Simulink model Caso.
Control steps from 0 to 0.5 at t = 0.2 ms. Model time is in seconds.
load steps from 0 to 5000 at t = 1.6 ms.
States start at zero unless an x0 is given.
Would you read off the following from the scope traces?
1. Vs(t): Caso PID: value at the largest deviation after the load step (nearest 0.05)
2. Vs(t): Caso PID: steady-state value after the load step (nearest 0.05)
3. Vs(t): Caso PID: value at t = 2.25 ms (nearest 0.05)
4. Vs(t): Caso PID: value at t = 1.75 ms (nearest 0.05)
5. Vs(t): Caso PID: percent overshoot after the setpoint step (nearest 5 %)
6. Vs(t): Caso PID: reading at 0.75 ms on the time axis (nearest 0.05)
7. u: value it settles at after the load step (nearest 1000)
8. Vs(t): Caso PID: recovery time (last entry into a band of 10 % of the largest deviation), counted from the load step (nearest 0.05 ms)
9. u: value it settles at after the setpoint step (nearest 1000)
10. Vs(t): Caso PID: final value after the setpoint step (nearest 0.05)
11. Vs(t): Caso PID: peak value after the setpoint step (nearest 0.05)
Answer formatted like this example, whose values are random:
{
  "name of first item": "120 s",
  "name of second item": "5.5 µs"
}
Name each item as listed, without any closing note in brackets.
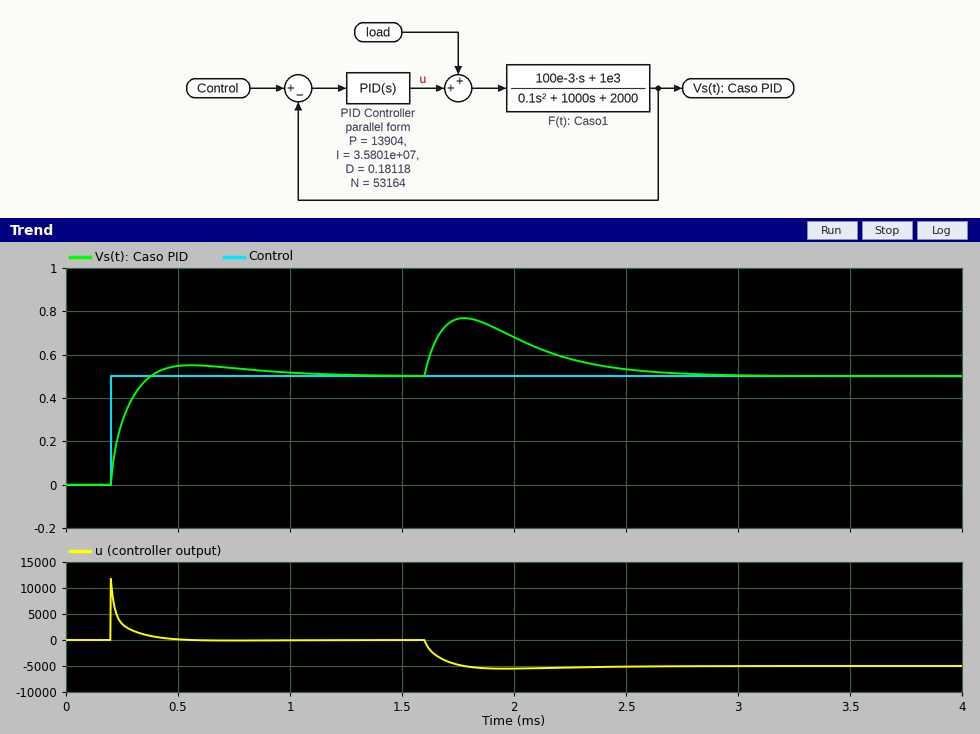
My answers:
{
  "Vs(t): Caso PID: value at the largest deviation after the load step": "0.75",
  "Vs(t): Caso PID: steady-state value after the load step": "0.50",
  "Vs(t): Caso PID: value at t = 2.25 ms": "0.60",
  "Vs(t): Caso PID: value at t = 1.75 ms": "0.75",
  "Vs(t): Caso PID: percent overshoot after the setpoint step": "10 %",
  "Vs(t): Caso PID: reading at 0.75 ms on the time axis": "0.55",
  "u: value it settles at after the load step": "-5000",
  "Vs(t): Caso PID: recovery time (last entry into a band of 10 % of the largest deviation), counted from the load step": "0.95 ms",
  "u: value it settles at after the setpoint step": "0",
  "Vs(t): Caso PID: final value after the setpoint step": "0.50",
  "Vs(t): Caso PID: peak value after the setpoint step": "0.55"
}
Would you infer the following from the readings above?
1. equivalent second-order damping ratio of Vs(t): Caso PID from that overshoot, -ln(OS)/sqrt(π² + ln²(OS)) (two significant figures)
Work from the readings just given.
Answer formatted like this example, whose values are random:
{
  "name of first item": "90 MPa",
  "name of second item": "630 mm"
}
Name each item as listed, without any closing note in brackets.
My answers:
{
  "equivalent second-order damping ratio of Vs(t): Caso PID from that overshoot, -ln(OS)/sqrt(π² + ln²(OS))": "0.59"
}
